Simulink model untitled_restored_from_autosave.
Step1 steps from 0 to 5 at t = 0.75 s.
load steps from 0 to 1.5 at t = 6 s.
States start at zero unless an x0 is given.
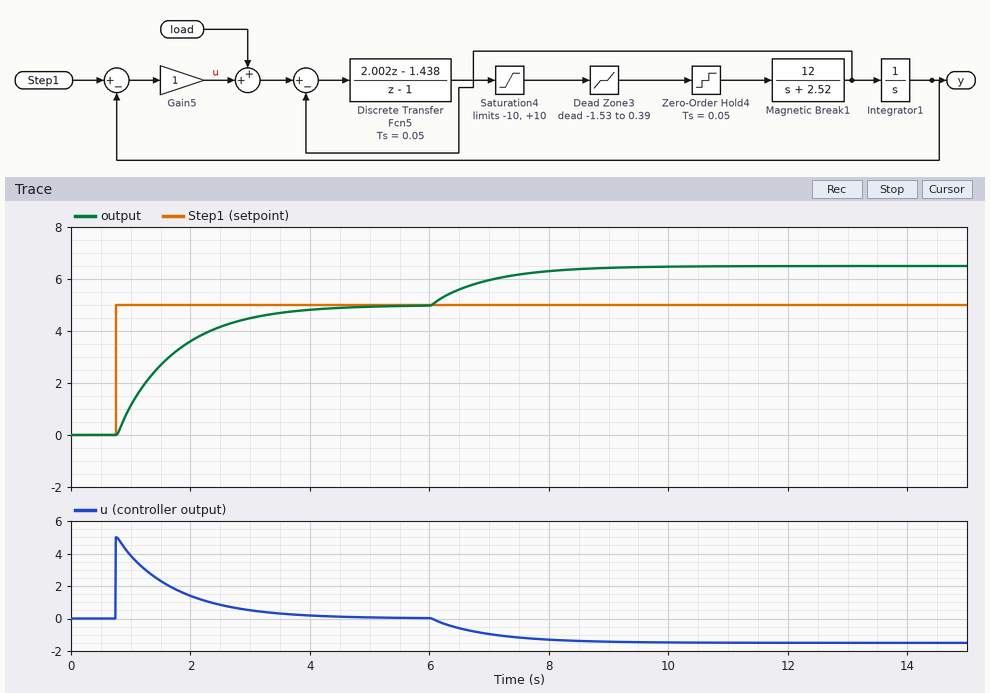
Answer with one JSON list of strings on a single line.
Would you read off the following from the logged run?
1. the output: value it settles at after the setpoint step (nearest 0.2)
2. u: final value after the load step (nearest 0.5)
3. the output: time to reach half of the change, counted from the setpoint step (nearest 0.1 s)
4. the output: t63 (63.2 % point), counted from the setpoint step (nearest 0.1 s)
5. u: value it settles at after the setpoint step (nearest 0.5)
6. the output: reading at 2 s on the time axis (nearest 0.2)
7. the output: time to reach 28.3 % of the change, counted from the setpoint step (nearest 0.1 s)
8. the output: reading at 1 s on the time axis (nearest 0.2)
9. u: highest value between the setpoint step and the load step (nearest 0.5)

["5.0", "-1.5", "0.7 s", "1.0 s", "0.0", "3.6", "0.3 s", "1.2", "5.0"]
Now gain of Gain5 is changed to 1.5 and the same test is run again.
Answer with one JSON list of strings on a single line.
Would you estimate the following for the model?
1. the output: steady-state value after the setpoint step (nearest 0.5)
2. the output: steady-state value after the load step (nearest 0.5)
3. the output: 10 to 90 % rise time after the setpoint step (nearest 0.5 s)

["5.0", "6.0", "1.5 s"]
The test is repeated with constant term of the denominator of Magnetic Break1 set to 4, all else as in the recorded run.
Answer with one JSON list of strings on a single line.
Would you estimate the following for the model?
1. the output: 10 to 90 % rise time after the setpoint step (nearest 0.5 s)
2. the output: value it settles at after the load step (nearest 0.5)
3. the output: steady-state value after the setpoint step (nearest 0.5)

["2.0 s", "6.5", "5.0"]
